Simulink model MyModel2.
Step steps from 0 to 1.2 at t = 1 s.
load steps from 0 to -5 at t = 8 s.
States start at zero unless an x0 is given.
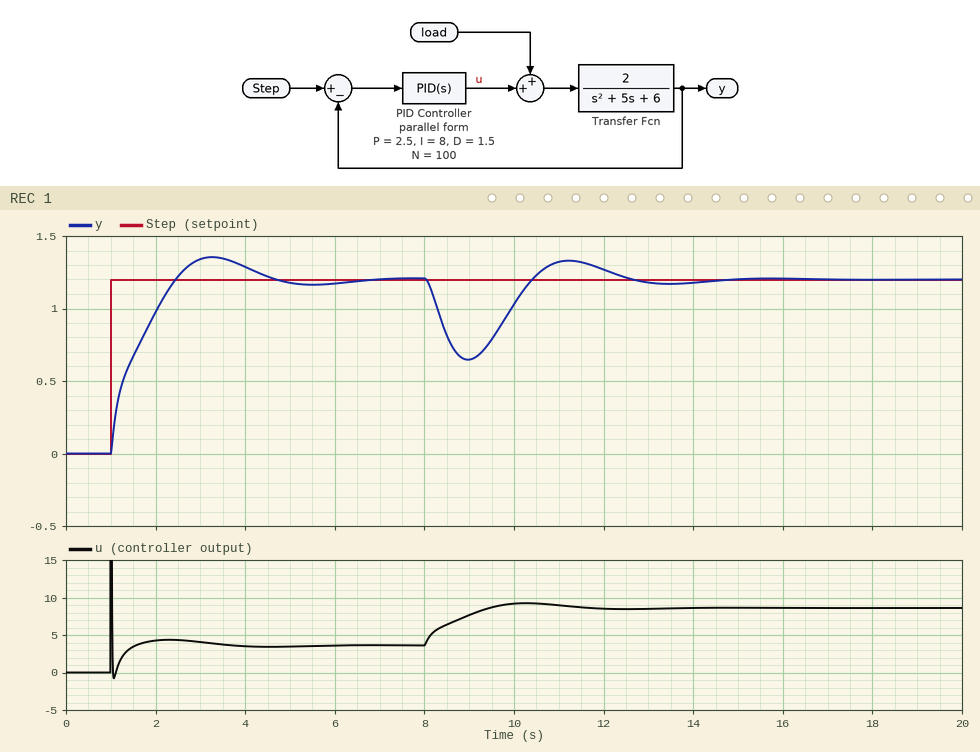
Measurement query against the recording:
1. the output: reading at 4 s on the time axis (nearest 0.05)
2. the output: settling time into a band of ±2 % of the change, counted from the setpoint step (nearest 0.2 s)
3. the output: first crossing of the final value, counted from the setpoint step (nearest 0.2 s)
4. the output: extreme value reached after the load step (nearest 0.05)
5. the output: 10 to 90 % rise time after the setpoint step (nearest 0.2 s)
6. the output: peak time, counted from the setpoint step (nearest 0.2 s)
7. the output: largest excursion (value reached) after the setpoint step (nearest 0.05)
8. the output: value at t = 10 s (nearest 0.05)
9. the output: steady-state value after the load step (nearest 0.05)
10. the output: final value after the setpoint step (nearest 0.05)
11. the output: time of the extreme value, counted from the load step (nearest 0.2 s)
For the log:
1.30
5.2 s
1.4 s
0.65
1.2 s
2.2 s
1.35
1.05
1.20
1.20
1.0 s
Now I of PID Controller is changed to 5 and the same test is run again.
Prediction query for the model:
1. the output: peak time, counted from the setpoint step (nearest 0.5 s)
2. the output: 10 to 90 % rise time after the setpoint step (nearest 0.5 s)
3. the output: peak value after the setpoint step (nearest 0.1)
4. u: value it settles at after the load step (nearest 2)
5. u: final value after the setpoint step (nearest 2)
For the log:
3.0 s
1.5 s
1.3
8
4
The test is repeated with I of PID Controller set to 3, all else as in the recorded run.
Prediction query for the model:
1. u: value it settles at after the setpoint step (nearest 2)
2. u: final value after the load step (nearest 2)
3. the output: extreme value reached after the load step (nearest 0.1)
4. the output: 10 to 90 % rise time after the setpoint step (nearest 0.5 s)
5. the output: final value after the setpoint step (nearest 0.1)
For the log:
4
8
0.5
2.5 s
1.2
